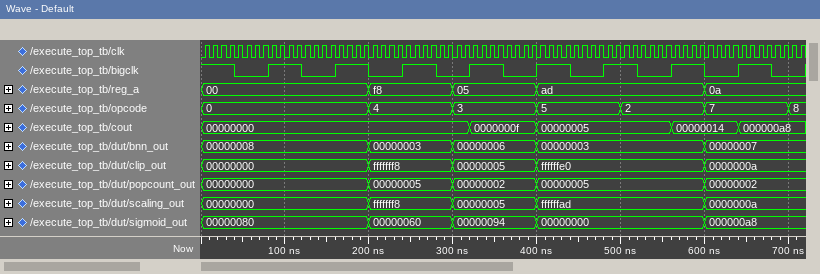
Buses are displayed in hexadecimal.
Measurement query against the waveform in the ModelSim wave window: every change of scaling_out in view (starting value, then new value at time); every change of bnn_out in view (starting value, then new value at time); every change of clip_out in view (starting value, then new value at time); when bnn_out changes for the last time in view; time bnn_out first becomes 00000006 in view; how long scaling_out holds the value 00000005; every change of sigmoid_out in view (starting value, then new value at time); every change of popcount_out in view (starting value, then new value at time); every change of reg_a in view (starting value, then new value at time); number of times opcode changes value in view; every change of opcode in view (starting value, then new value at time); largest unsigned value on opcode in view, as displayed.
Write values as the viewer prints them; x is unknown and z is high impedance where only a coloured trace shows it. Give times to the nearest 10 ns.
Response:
00000000, fffffff8 at 200 ns, 00000005 at 300 ns, ffffffad at 400 ns, 0000000a at 600 ns
00000008, 00000003 at 200 ns, 00000006 at 300 ns, 00000003 at 400 ns, 00000007 at 600 ns
00000000, fffffff8 at 200 ns, 00000005 at 300 ns, ffffffe0 at 400 ns, 0000000a at 600 ns
600 ns
300 ns
100 ns
00000080, 00000060 at 200 ns, 00000094 at 300 ns, 00000000 at 400 ns, 000000a8 at 600 ns
00000000, 00000005 at 200 ns, 00000002 at 300 ns, 00000005 at 400 ns, 00000002 at 600 ns
00, f8 at 200 ns, 05 at 300 ns, ad at 400 ns, 0a at 600 ns
6
0, 4 at 200 ns, 3 at 300 ns, 5 at 400 ns, 2 at 500 ns, 7 at 600 ns, 8 at 700 ns
8
